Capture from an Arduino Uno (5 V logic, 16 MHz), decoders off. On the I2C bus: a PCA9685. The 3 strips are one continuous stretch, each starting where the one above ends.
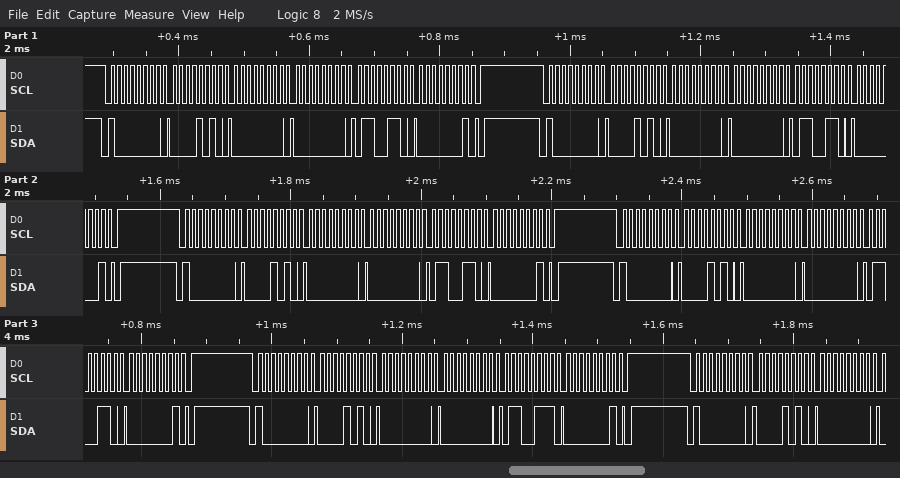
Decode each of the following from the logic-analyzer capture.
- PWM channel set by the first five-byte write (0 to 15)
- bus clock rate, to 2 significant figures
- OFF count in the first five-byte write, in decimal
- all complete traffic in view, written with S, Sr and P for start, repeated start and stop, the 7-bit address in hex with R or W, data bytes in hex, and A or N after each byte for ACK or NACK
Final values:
1
100 kHz
358
S 40W A 0A A 00 A 00 A 66 A 01 A P S 40W A 0A A 00 A 00 A 66 A 01 A P S 40W A 0A A 00 A 00 A 66 A 01 A P S 40W A 0A A 00 A 00 A 66 A 01 A P S 40W A 0A A 00 A 00 A 67 A 01 A P S 40W A 0A A 00 A
